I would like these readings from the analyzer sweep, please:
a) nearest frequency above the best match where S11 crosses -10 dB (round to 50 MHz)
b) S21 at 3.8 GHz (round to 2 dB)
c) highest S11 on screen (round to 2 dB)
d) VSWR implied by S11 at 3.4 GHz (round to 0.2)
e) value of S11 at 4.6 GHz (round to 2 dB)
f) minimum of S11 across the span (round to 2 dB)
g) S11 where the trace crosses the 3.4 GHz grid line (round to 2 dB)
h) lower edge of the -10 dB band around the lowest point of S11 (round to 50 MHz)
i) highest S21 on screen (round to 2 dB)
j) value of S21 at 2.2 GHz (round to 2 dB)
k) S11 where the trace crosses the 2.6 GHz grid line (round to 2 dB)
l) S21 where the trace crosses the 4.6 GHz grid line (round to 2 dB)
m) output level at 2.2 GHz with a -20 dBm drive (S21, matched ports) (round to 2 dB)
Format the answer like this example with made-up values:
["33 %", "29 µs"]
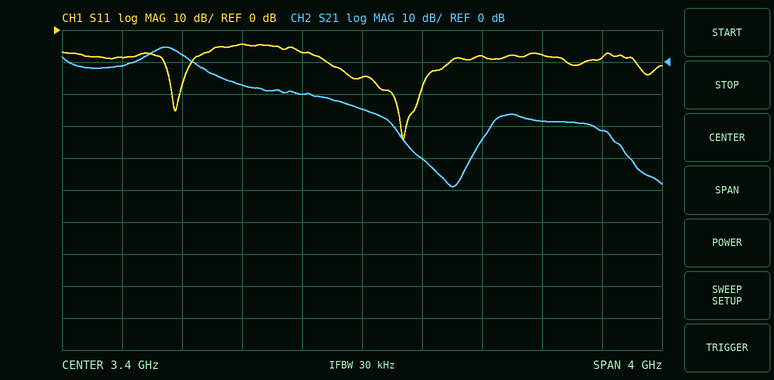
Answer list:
["4.00 GHz", "-30 dB", "-4 dB", "1.4", "-8 dB", "-34 dB", "-14 dB", "3.15 GHz", "4 dB", "2 dB", "-4 dB", "-18 dB", "-18 dBm"]
